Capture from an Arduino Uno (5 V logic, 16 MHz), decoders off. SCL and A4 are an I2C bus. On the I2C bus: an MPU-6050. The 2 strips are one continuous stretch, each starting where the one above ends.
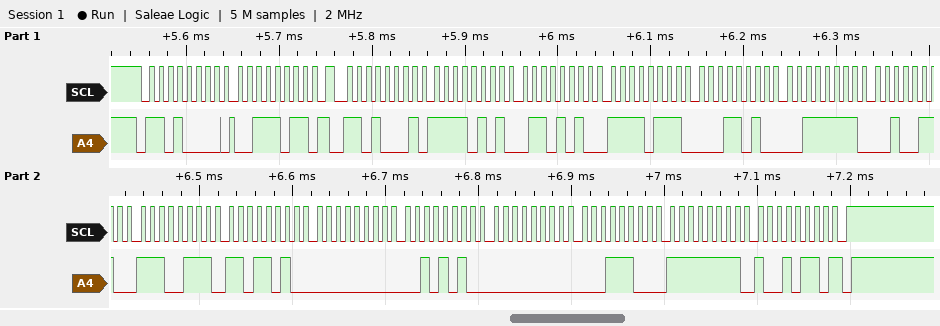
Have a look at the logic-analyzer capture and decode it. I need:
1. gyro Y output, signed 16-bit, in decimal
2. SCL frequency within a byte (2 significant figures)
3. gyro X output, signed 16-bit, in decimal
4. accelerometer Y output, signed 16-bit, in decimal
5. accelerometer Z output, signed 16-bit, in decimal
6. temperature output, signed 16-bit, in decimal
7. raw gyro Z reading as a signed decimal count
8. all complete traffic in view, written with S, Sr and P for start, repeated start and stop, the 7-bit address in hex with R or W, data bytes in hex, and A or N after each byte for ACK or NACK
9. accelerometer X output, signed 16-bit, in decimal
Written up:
28
100 kHz
42
-2278
16166
-6182
-106
S 68W A 3B A Sr 68R A F5 A 6A A F7 A 1A A 3F A 26 A E7 A DA A 00 A 2A A 00 A 1C A FF A 96 N P
-2710
